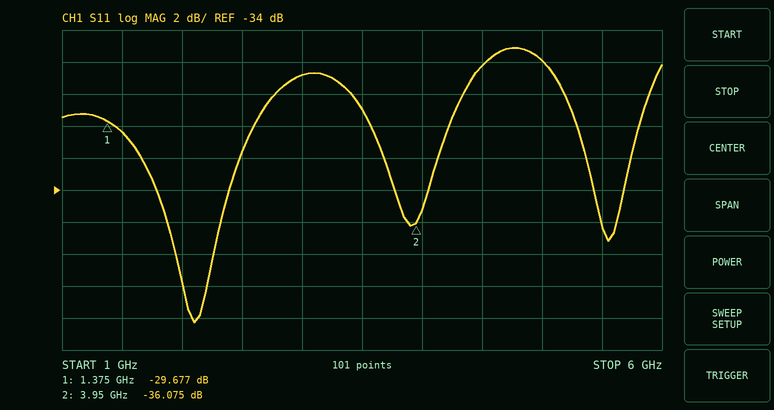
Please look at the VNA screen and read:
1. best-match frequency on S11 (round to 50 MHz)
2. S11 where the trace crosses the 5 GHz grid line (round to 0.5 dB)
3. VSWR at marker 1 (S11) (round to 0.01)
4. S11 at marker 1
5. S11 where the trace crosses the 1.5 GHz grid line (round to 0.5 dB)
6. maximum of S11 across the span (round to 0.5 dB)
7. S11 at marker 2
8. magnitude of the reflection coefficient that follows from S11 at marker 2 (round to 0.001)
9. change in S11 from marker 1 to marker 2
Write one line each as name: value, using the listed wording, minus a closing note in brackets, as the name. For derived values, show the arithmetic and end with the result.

best-match frequency on S11: 2.10 GHz
S11 where the trace crosses the 5 GHz grid line: -26.0 dB
VSWR at marker 1 (S11): (1 + 0.0328)/(1 − 0.0328) ≈ 1.07
S11 at marker 1: -29.677 dB
S11 where the trace crosses the 1.5 GHz grid line: -30.5 dB
maximum of S11 across the span: -25.0 dB
S11 at marker 2: -36.075 dB
magnitude of the reflection coefficient that follows from S11 at marker 2: 10^(-36.075/20) ≈ 0.016
change in S11 from marker 1 to marker 2: -36.075 − (-29.677) = -6.398 dB
